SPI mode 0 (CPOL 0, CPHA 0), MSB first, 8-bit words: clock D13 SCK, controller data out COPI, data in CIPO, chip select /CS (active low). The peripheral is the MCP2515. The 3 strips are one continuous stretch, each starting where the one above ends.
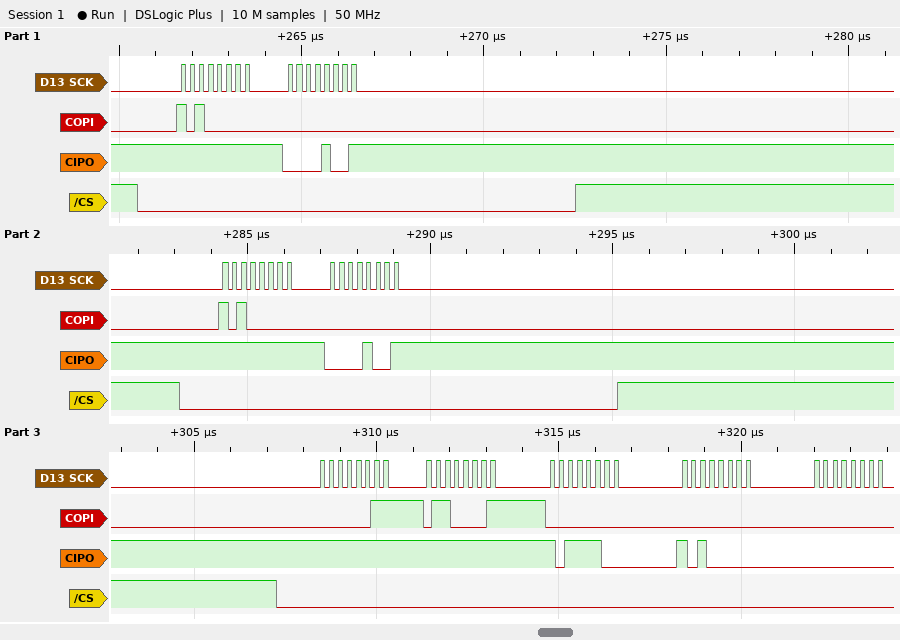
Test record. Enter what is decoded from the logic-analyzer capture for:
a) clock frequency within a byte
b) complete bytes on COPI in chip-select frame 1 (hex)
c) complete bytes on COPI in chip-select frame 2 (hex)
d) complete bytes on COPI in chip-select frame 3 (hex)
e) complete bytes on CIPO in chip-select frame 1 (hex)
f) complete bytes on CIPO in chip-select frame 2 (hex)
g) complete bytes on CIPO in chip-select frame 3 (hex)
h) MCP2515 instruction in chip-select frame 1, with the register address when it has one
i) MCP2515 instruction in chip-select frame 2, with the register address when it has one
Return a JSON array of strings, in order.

["4 MHz", "A0 00", "A0 00", "03 61 00 00 00", "FF 09", "FF 09", "FF FF BC A0 00", "READ STATUS", "READ STATUS"]
